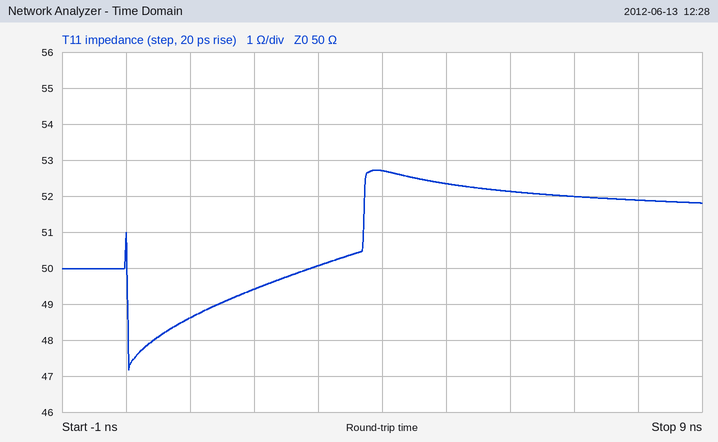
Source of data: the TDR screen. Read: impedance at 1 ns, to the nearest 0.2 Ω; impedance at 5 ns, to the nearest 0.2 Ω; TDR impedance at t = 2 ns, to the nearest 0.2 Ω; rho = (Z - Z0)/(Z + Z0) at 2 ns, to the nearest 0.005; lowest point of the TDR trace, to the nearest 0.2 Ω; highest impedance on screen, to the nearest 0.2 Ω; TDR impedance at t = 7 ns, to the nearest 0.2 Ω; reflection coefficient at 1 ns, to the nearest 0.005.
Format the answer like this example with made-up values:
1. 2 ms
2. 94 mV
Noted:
1. 48.6 Ω
2. 52.4 Ω
3. 49.4 Ω
4. -0.005
5. 47.2 Ω
6. 52.8 Ω
7. 52.0 Ω
8. -0.015
